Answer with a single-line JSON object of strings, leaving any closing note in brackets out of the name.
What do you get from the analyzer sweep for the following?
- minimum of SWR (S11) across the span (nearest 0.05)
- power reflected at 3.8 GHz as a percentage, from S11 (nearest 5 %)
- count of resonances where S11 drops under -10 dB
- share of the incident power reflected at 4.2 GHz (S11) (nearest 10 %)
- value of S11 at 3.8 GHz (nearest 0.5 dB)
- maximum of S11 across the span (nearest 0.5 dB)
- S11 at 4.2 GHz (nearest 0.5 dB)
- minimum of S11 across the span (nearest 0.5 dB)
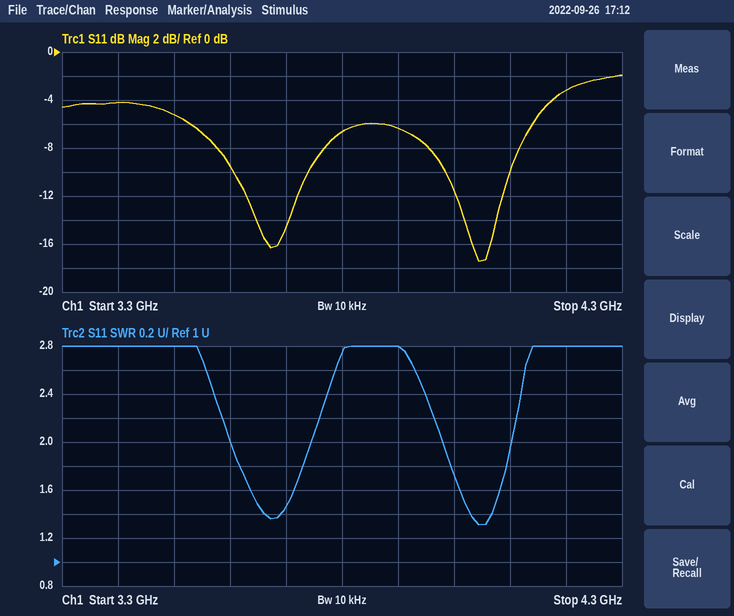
{"minimum of SWR (S11) across the span": "1.30", "power reflected at 3.8 GHz as a percentage, from S11": "20 %", "count of resonances where S11 drops under -10 dB": "2", "share of the incident power reflected at 4.2 GHz (S11)": "50 %", "value of S11 at 3.8 GHz": "-6.5 dB", "maximum of S11 across the span": "-2.0 dB", "S11 at 4.2 GHz": "-3.0 dB", "minimum of S11 across the span": "-17.5 dB"}
